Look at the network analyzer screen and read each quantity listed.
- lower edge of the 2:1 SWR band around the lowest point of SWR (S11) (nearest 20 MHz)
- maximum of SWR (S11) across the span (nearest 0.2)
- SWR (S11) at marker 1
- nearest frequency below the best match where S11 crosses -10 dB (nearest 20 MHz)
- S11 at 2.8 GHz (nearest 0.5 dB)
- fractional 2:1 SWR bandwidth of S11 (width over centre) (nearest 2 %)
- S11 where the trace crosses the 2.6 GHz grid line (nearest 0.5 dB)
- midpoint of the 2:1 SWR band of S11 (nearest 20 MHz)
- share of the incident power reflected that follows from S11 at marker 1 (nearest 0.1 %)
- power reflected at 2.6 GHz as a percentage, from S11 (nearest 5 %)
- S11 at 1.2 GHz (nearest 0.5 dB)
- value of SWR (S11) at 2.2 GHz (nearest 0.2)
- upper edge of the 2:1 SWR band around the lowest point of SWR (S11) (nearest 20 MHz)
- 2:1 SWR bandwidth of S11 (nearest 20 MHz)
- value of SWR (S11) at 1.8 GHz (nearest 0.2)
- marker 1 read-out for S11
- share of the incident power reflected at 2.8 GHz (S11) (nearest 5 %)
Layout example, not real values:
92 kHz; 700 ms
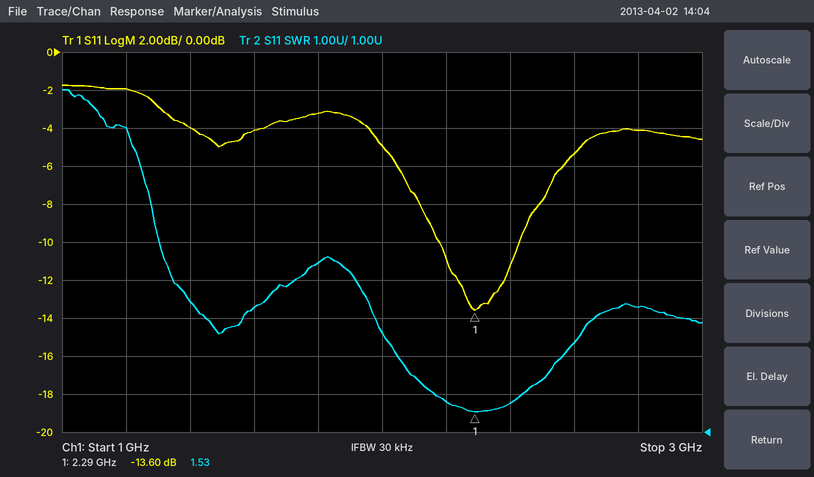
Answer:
2.16 GHz; 10.0; 1.53; 2.18 GHz; -4.0 dB; 12 %; -5.5 dB; 2.30 GHz; 4.4 %; 30 %; -2.0 dB; 1.8; 2.44 GHz; 280 MHz; 5.4; -13.60 dB; 40 %
